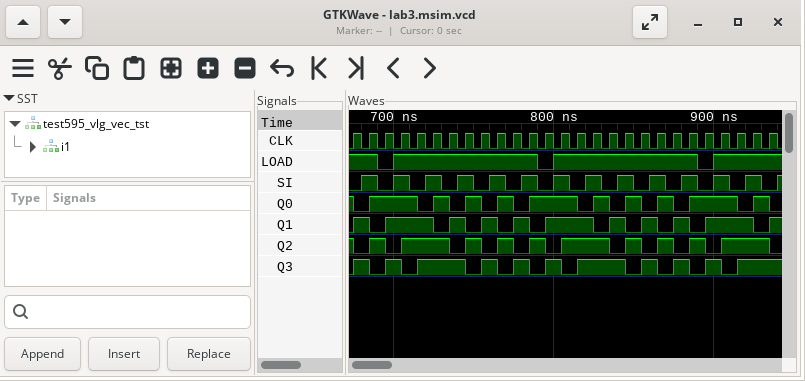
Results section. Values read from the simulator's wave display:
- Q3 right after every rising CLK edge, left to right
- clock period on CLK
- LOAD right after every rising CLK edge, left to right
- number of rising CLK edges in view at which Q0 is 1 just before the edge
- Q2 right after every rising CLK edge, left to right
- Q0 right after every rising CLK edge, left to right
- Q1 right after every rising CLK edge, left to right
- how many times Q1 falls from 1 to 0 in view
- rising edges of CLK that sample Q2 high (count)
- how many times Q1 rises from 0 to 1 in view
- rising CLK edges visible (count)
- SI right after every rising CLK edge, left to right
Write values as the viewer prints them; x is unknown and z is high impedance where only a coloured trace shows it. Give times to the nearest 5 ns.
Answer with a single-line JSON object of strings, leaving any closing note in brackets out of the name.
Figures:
{"Q3 right after every rising CLK edge, left to right": "1 0 1 0 1 1 1 0 1 0 1 0 1 0 1 1 1 0 1 0 1 0 1 0 1 1 1", "clock period on CLK": "10 ns", "LOAD right after every rising CLK edge, left to right": "1 1 0 1 1 1 1 1 1 1 1 1 0 1 1 1 1 1 1 1 1 1 0 1 1 1 1", "number of rising CLK edges in view at which Q0 is 1 just before the edge": "17", "Q2 right after every rising CLK edge, left to right": "0 1 0 1 1 1 0 1 0 1 0 1 0 1 1 1 0 1 0 1 0 1 0 1 1 1 0", "Q0 right after every rising CLK edge, left to right": "0 1 1 1 0 1 0 1 0 1 0 1 1 1 0 1 0 1 0 1 0 1 1 1 0 1 0", "Q1 right after every rising CLK edge, left to right": "1 0 1 1 1 0 1 0 1 0 1 0 1 1 1 0 1 0 1 0 1 0 1 1 1 0 1", "how many times Q1 falls from 1 to 0 in view": "10", "rising edges of CLK that sample Q2 high": "17", "how many times Q1 rises from 0 to 1 in view": "11", "rising CLK edges visible": "27", "SI right after every rising CLK edge, left to right": "0 1 0 1 0 1 0 1 0 1 0 1 0 1 0 1 0 1 0 1 0 1 0 1 0 1 0"}
